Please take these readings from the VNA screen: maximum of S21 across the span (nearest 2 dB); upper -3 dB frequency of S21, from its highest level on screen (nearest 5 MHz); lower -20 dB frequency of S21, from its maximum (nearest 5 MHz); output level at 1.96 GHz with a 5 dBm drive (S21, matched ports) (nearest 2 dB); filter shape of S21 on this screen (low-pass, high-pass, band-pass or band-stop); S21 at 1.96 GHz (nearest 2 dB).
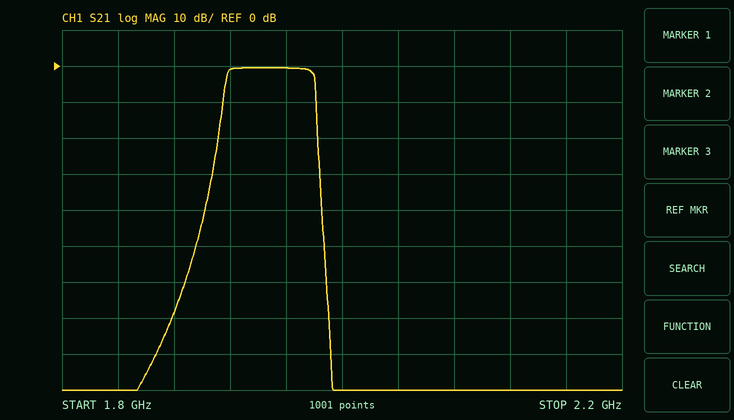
0 dB
1.980 GHz
1.910 GHz
4 dBm
band-pass
0 dB
